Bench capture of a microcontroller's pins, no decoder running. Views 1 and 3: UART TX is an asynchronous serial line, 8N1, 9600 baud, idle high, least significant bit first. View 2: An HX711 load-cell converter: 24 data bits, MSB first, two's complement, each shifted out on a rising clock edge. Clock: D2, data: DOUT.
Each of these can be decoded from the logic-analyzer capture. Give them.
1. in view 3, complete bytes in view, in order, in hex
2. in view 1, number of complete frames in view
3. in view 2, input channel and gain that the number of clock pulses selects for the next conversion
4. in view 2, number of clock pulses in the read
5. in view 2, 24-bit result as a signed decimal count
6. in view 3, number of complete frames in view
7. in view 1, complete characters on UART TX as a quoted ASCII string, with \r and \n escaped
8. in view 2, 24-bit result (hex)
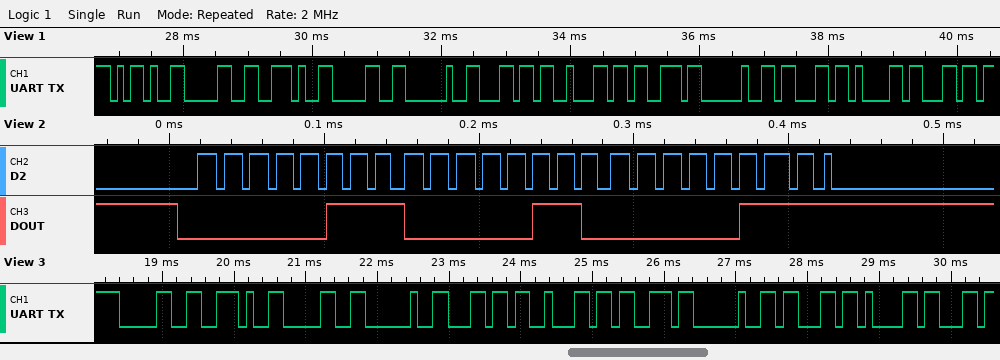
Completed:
0x30 0x2E 0x30 0x20 0x6C 0x62 0x73 0x20 0x63 0x61
12
channel A, gain 128
25
460295
10
"-0.0 lbs cal"
0x070607
